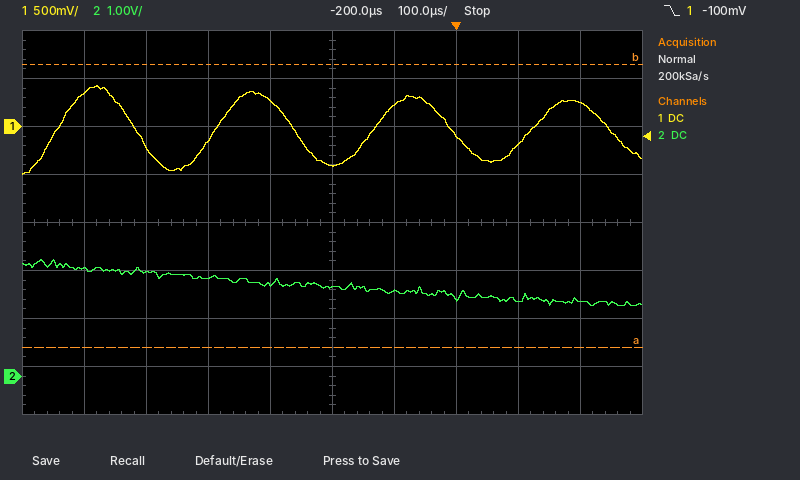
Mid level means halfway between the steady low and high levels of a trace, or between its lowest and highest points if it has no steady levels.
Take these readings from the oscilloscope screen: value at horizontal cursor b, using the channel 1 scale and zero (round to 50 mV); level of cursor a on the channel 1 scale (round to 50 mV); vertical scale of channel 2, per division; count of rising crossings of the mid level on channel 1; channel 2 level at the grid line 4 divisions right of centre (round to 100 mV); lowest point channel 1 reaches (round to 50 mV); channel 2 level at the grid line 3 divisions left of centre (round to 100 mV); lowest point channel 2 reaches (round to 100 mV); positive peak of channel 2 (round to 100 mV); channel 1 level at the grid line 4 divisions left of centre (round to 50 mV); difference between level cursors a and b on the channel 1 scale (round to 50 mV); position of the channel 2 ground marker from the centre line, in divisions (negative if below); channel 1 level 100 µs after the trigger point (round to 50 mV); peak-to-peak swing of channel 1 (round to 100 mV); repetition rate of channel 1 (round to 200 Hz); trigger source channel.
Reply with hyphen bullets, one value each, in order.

- 650 mV
- -2.30 V
- 1 V
- 4
- 1.6 V
- -500 mV
- 2.2 V
- 1.5 V
- 2.4 V
- 350 mV
- 2.95 V
- -3.2 div
- -200 mV
- 900 mV
- 4.0 kHz
- channel 1
